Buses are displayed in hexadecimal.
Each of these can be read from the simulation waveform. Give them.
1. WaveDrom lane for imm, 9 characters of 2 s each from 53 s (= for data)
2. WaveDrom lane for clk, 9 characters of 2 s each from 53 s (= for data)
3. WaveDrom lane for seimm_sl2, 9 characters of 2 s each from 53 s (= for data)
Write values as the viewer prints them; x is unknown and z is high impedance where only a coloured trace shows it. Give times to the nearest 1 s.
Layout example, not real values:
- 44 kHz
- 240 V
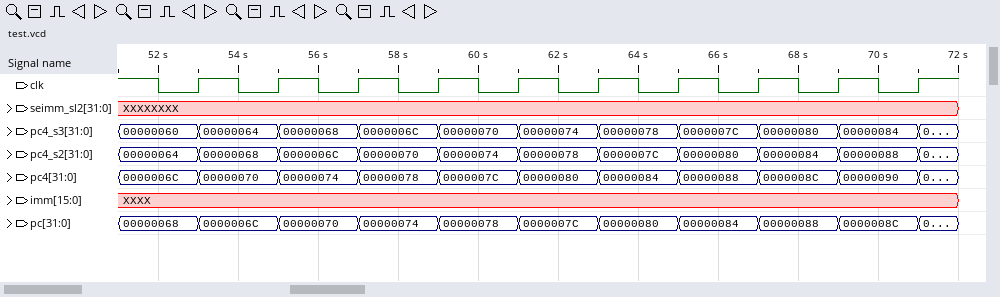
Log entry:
- {name: 'imm', wave: 'x........'}
- {name: 'clk', wave: 'p........'}
- {name: 'seimm_sl2', wave: '=........', data: 'XXXXXXXX'}
